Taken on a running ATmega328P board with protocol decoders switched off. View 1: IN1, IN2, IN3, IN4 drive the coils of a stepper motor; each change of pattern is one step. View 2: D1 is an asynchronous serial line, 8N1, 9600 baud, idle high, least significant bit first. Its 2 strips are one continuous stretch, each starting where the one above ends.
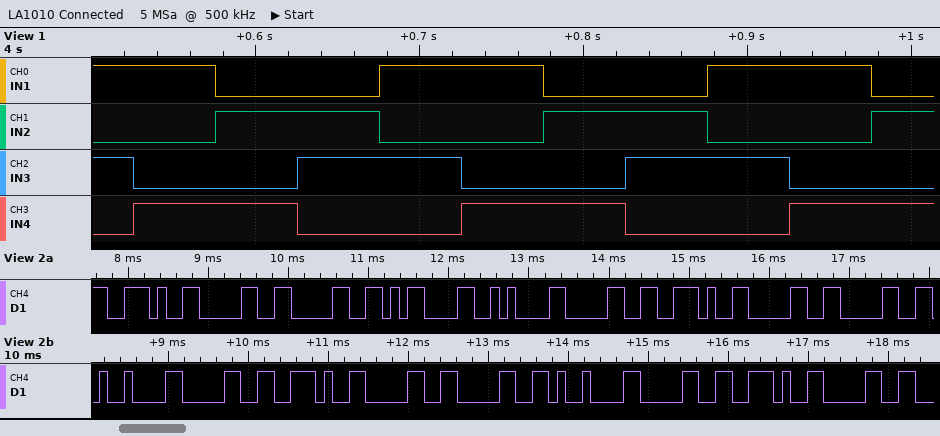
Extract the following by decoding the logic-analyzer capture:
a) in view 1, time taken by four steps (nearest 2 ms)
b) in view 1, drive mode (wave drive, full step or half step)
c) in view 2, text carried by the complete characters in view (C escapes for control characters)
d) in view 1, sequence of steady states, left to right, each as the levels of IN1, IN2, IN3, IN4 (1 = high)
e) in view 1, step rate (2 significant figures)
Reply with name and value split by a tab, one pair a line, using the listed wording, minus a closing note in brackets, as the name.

in view 1, time taken by four steps	200 ms
in view 1, drive mode	full step
in view 2, text carried by the complete characters in view	".00\r\n0.00\t0.00\t0.0"
in view 1, sequence of steady states, left to right, each as the levels of IN1, IN2, IN3, IN4	1010 1001 0101 0110 1010 1001 0101 0110 1010 1001 0101
in view 1, step rate	20 steps/s
